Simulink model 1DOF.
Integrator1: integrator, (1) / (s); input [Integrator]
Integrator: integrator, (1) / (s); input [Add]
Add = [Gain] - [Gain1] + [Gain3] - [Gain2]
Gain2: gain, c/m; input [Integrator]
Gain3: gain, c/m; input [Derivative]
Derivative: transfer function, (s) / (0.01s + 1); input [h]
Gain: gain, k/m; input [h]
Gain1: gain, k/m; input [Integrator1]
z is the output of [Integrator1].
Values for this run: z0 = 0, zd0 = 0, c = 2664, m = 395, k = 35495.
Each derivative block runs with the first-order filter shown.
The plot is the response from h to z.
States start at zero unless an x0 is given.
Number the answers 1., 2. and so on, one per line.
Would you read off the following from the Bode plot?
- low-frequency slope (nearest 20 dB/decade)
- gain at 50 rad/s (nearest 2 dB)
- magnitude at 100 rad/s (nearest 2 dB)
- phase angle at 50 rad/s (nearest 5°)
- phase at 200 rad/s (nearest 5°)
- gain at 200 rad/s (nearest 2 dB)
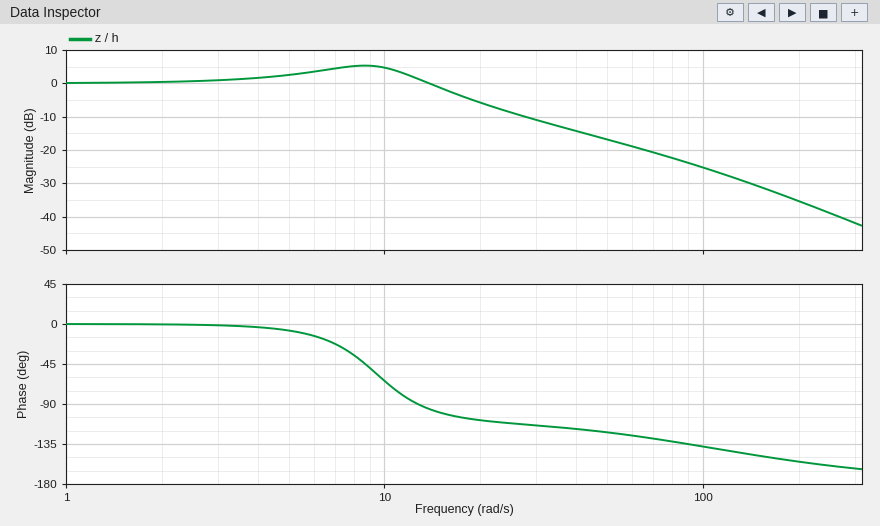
1. 0 dB/decade
2. -16 dB
3. -26 dB
4. -120°
5. -155°
6. -36 dB
